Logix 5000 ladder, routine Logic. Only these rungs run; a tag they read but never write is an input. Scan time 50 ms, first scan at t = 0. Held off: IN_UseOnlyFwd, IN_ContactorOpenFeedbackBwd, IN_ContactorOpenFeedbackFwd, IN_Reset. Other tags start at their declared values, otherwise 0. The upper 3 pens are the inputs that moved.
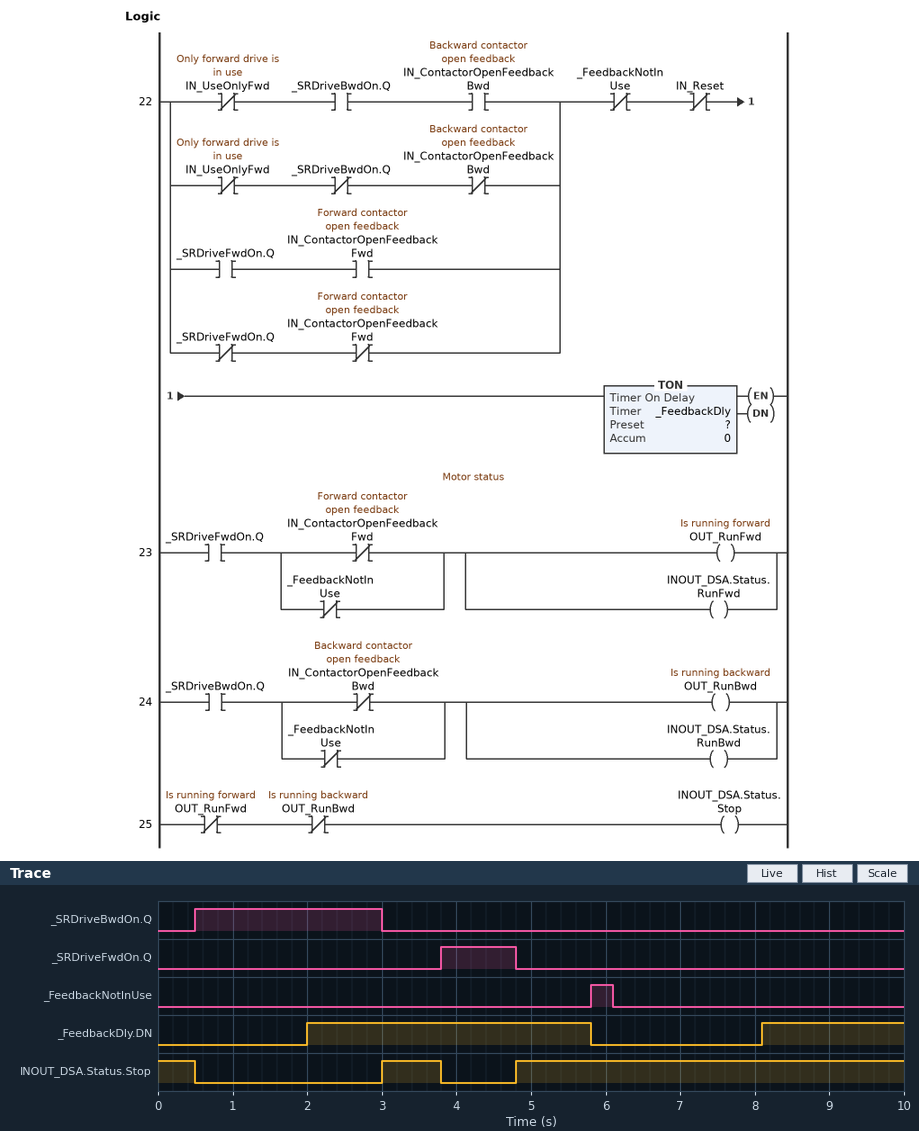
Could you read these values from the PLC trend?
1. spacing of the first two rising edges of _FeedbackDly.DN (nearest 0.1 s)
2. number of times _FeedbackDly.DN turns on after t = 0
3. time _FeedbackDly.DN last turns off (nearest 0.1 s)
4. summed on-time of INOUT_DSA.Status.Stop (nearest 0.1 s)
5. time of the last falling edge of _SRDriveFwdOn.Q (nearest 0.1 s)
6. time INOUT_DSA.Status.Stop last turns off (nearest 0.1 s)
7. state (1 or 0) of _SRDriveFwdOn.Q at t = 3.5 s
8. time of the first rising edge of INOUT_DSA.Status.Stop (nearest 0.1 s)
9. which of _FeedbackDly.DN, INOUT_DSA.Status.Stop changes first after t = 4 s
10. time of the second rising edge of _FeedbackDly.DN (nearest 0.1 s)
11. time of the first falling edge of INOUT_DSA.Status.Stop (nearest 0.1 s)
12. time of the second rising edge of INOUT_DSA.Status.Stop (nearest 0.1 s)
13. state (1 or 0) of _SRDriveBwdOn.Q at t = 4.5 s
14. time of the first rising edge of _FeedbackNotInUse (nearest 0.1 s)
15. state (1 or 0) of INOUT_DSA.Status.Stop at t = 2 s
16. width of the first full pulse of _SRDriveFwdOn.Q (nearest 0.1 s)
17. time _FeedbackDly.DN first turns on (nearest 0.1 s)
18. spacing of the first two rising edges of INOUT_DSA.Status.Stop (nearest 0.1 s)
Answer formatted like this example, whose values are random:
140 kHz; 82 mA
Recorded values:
6.1 s; 2; 5.8 s; 6.5 s; 4.8 s; 3.8 s; 0; 3.0 s; INOUT_DSA.Status.Stop; 8.1 s; 0.5 s; 4.8 s; 0; 5.8 s; 0; 1.0 s; 2.0 s; 1.8 s
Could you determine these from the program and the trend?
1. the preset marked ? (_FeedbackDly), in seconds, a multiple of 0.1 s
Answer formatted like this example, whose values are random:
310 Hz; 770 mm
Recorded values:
2.0 s
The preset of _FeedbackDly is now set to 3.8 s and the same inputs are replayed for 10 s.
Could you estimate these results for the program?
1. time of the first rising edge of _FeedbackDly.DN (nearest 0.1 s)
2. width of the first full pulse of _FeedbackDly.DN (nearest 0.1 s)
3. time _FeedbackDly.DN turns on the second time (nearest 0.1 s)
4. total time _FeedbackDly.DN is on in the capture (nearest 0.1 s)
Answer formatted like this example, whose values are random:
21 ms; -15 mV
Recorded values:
3.8 s; 2.0 s; 9.9 s; 2.1 s
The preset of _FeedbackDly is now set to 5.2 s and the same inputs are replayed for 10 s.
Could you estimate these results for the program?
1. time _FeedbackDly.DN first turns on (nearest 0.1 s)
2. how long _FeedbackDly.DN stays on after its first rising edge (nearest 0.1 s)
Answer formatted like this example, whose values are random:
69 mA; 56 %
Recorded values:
5.2 s; 0.6 s
